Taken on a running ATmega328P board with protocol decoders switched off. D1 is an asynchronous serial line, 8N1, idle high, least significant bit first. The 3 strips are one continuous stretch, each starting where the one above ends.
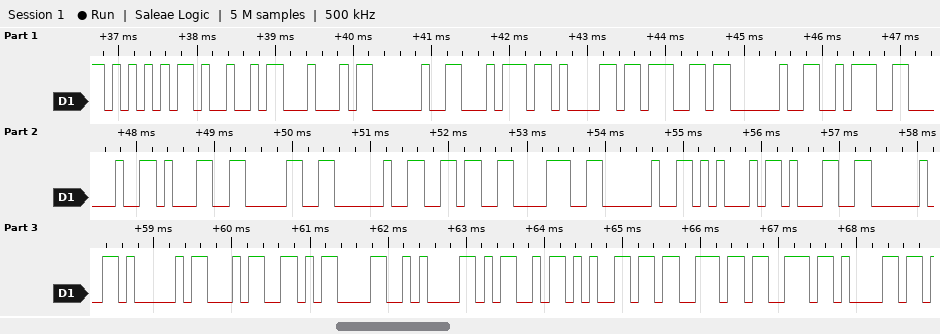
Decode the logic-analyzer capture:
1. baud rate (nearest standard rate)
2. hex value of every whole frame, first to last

9600 baud
55 49 44 20 74 61 67 20 3A 20 31 30 20 36 38 20 45 31 20 41 34 0D 0A 4D 65 73 73 61
